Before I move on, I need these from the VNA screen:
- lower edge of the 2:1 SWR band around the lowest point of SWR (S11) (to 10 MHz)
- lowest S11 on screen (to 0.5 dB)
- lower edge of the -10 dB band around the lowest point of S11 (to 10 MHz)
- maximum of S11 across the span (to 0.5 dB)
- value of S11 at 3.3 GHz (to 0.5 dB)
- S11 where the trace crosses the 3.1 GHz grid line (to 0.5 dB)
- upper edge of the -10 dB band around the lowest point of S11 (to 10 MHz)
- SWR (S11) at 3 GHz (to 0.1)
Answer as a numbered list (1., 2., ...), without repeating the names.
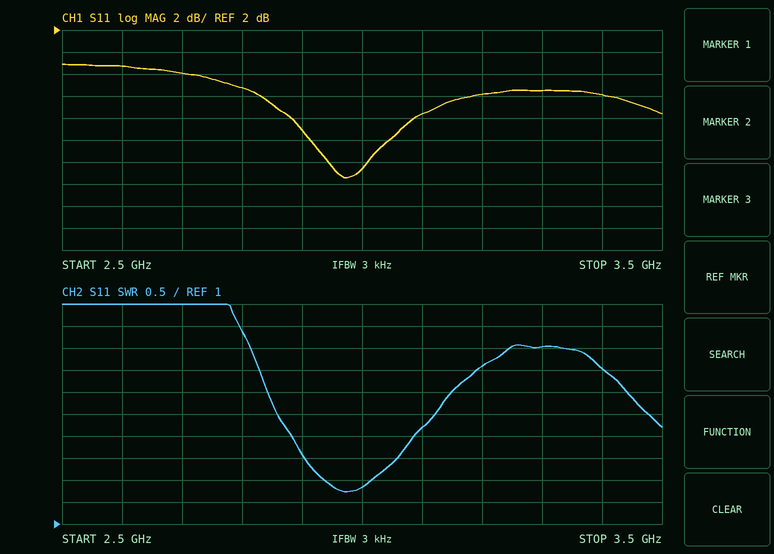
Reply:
1. 2.94 GHz
2. -11.5 dB
3. 2.94 GHz
4. -1.0 dB
5. -3.5 dB
6. -5.5 dB
7. 3.01 GHz
8. 1.8
